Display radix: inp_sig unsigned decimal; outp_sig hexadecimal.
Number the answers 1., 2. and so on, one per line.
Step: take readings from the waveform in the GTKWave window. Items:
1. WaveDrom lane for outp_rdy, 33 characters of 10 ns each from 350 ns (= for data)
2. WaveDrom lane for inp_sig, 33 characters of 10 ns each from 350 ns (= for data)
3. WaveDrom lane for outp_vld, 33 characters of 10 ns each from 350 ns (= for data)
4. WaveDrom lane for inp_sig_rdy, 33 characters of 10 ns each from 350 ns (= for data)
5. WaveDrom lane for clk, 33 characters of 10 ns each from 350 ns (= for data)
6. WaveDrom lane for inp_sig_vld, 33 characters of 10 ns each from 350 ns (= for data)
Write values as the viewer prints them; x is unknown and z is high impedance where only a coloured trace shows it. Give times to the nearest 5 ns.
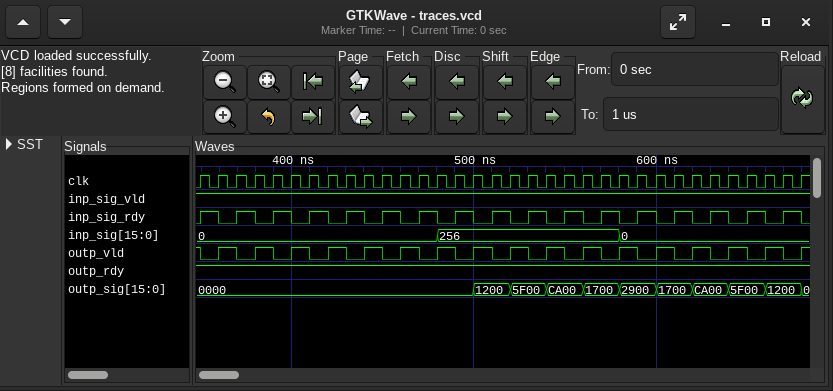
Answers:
1. {name: 'outp_rdy', wave: '1................................'}
2. {name: 'inp_sig', wave: '=............=.........=.........', data: '0 256 0'}
3. {name: 'outp_vld', wave: '010101010101010101010101010101010'}
4. {name: 'inp_sig_rdy', wave: '101010101010101010101010101010101'}
5. {name: 'clk', wave: 'p................................'}
6. {name: 'inp_sig_vld', wave: '1................................'}
